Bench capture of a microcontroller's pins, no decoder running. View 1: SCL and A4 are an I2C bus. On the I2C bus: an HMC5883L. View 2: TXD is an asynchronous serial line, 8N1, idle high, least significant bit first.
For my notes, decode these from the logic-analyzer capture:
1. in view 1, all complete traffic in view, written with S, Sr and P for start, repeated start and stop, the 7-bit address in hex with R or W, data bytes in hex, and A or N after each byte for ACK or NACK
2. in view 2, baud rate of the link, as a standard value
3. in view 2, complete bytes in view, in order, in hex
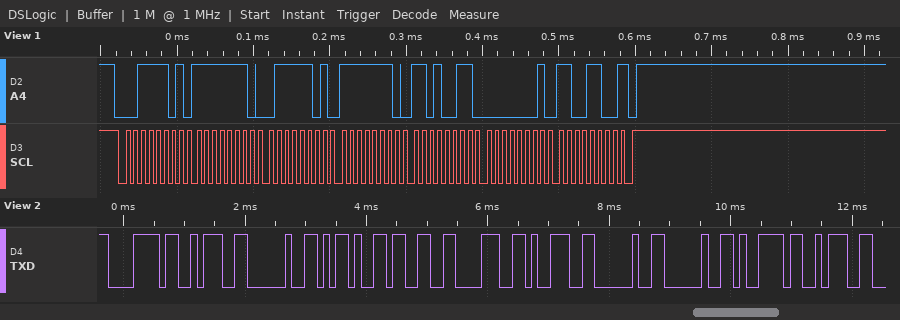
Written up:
S 1ER A FE A 7D A FE A D3 A 01 A CC N P
9600 baud
78 3A 20 2D 33 38 39 20 20 79 3A
